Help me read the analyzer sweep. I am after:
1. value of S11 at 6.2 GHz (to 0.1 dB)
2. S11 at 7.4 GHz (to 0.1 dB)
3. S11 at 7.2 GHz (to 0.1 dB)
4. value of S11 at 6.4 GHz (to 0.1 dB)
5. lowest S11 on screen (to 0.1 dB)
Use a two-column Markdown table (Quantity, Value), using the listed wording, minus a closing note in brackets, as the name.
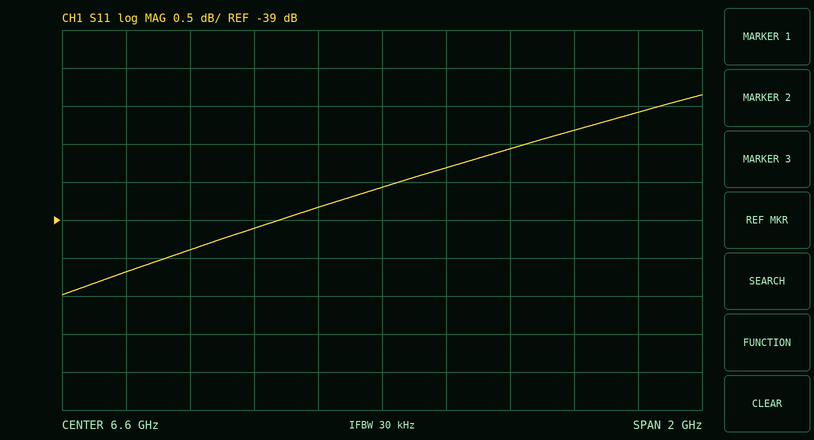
| Quantity | Value |
|---|---|
| value of S11 at 6.2 GHz | -39.1 dB |
| S11 at 7.4 GHz | -37.6 dB |
| S11 at 7.2 GHz | -37.8 dB |
| value of S11 at 6.4 GHz | -38.8 dB |
| lowest S11 on screen | -40.0 dB |
